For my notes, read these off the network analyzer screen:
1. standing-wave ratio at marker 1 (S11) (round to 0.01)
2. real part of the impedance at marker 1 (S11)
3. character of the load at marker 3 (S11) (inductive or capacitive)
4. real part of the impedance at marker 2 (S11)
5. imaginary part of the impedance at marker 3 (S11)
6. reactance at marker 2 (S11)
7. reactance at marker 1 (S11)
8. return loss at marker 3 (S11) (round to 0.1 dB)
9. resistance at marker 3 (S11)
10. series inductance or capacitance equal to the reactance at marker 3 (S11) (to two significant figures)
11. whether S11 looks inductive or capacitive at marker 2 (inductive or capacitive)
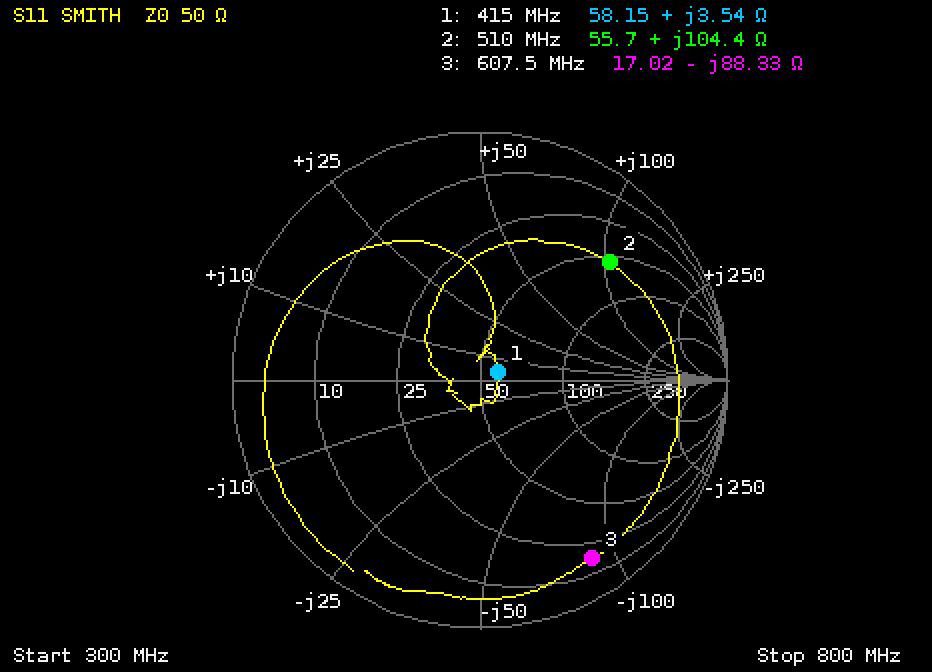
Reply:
1.18
58.15 Ω
capacitive
55.7 Ω
-88.33 Ω
+104.4 Ω
+3.54 Ω
1.4 dB
17.02 Ω
3.0 pF
inductive
